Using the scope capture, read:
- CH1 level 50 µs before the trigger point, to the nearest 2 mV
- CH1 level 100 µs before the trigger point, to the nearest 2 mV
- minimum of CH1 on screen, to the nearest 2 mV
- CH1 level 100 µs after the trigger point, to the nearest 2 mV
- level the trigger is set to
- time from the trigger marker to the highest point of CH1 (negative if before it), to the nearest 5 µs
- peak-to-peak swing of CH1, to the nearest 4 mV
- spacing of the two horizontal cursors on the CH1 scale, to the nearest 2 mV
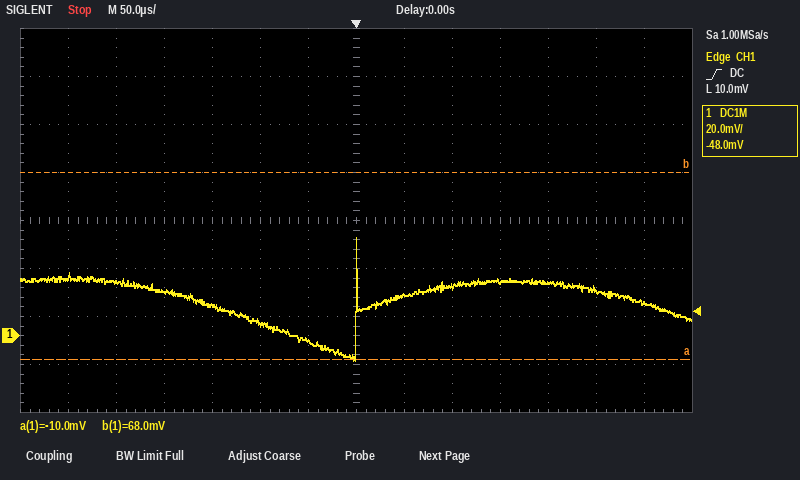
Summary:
-2 mV
6 mV
-10 mV
20 mV
10.0 mV
0 µs
52 mV
78 mV
